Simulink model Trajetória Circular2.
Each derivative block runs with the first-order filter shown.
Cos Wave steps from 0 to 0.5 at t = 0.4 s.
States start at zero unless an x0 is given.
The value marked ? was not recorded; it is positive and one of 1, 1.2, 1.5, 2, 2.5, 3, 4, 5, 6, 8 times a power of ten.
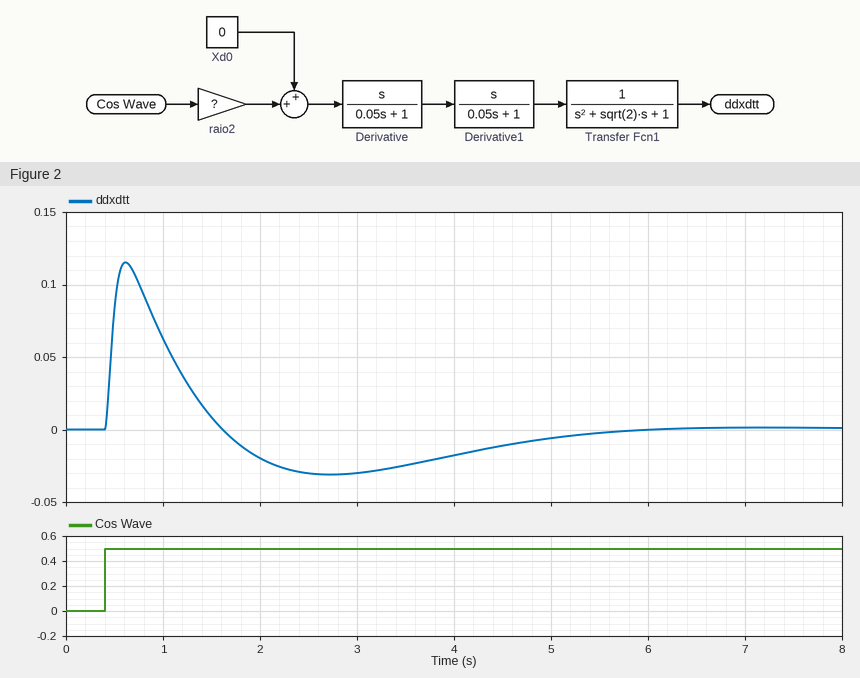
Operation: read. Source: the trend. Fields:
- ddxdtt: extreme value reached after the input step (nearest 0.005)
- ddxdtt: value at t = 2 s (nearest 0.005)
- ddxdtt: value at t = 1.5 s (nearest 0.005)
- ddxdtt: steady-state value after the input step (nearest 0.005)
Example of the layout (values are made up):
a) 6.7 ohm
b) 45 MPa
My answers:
a) 0.115
b) -0.020
c) 0.010
d) 0.000
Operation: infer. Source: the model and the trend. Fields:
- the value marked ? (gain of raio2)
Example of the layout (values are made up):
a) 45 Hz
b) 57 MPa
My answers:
a) 0.3
